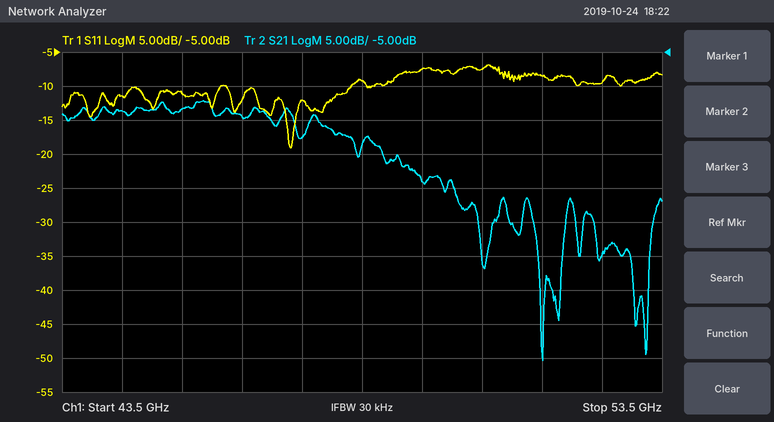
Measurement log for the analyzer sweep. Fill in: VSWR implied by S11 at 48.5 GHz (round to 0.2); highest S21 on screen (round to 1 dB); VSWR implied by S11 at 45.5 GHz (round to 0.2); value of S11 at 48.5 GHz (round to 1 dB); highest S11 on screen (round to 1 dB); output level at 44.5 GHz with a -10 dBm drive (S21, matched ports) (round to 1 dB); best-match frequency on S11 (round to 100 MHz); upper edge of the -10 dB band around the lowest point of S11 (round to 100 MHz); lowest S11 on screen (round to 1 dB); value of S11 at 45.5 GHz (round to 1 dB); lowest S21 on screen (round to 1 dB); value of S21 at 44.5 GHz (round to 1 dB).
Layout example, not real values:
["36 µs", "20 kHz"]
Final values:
["2.0", "-12 dB", "1.8", "-9 dB", "-7 dB", "-24 dBm", "47.3 GHz", "48.3 GHz", "-19 dB", "-11 dB", "-50 dB", "-14 dB"]
